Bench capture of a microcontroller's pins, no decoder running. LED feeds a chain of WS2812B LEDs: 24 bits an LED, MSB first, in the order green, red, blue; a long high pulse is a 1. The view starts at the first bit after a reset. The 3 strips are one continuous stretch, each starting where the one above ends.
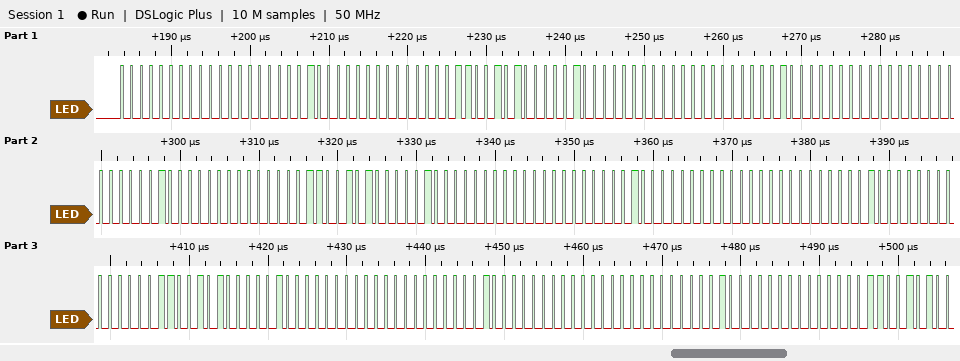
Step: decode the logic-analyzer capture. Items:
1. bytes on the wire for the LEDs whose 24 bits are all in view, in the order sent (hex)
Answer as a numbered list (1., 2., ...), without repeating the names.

1. 00 00 10 00 32 82 00 00 10 00 00 10 00 32 82 00 00 10 00 00 10 00 32 82 00 00 10 00 00 10
